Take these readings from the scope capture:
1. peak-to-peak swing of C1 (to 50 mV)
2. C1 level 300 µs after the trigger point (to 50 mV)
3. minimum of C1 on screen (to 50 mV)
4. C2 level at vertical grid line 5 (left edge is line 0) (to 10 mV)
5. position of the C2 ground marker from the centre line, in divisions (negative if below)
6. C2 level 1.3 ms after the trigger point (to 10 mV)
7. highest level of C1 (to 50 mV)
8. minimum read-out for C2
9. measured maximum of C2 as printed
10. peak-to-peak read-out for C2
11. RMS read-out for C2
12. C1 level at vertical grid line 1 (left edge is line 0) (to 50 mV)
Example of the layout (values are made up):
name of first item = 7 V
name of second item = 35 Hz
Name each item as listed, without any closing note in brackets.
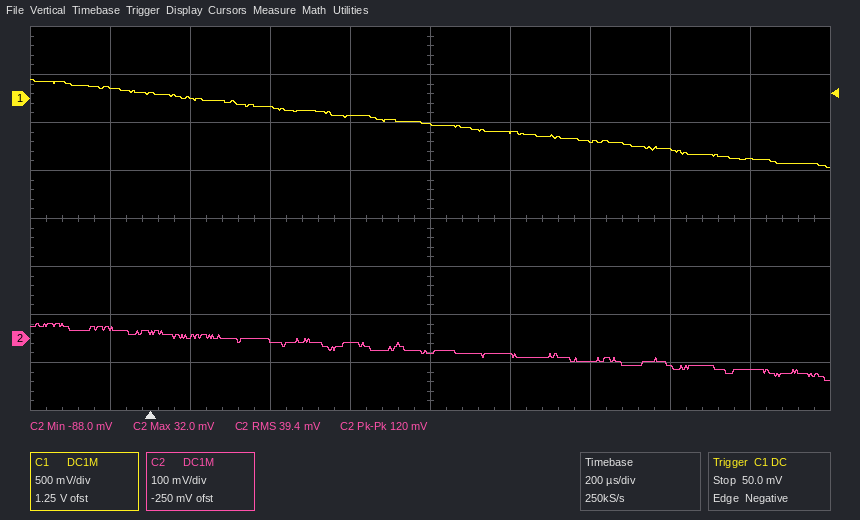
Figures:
peak-to-peak swing of C1 = 900 mV
C1 level 300 µs after the trigger point = -100 mV
minimum of C1 on screen = -700 mV
C2 level at vertical grid line 5 (left edge is line 0) = -30 mV
position of the C2 ground marker from the centre line, in divisions = -2.5 div
C2 level 1.3 ms after the trigger point = -60 mV
highest level of C1 = 200 mV
minimum read-out for C2 = -88.0 mV
measured maximum of C2 as printed = 32.0 mV
peak-to-peak read-out for C2 = 120 mV
RMS read-out for C2 = 39.4 mV
C1 level at vertical grid line 1 (left edge is line 0) = 100 mV
